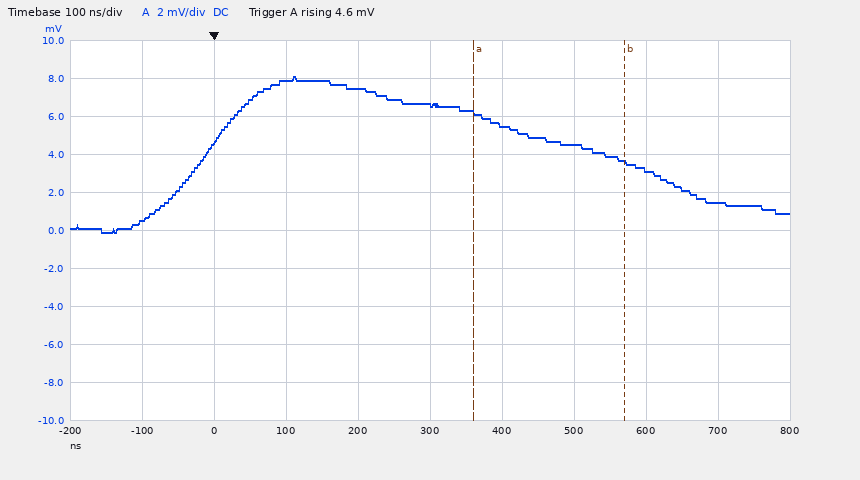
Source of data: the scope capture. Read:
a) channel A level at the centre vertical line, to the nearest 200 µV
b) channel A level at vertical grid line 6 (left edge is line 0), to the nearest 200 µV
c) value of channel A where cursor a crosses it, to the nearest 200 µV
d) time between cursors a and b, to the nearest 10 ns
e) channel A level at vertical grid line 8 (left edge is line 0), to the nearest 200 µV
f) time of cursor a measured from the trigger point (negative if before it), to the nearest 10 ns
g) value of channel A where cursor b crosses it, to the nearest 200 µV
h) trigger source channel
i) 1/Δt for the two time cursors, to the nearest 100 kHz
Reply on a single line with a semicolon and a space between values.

6.6 mV; 5.6 mV; 6.2 mV; 210 ns; 3.2 mV; +360 ns; 3.6 mV; channel A; 4.8 MHz
